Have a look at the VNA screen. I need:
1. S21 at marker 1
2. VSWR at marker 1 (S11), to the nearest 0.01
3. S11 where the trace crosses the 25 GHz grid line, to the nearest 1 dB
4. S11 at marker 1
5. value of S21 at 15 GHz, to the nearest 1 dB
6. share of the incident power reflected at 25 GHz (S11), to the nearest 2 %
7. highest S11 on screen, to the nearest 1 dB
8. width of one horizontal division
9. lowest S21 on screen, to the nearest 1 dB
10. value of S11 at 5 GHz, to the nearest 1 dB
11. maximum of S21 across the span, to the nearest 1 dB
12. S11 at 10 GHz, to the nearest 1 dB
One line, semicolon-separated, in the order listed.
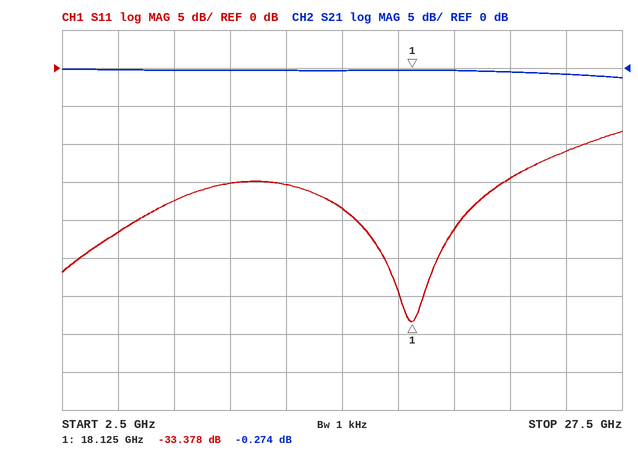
-0.274 dB; 1.04; -11 dB; -33.378 dB; 0 dB; 8 %; -8 dB; 2.5 GHz; -1 dB; -22 dB; 0 dB; -15 dB
